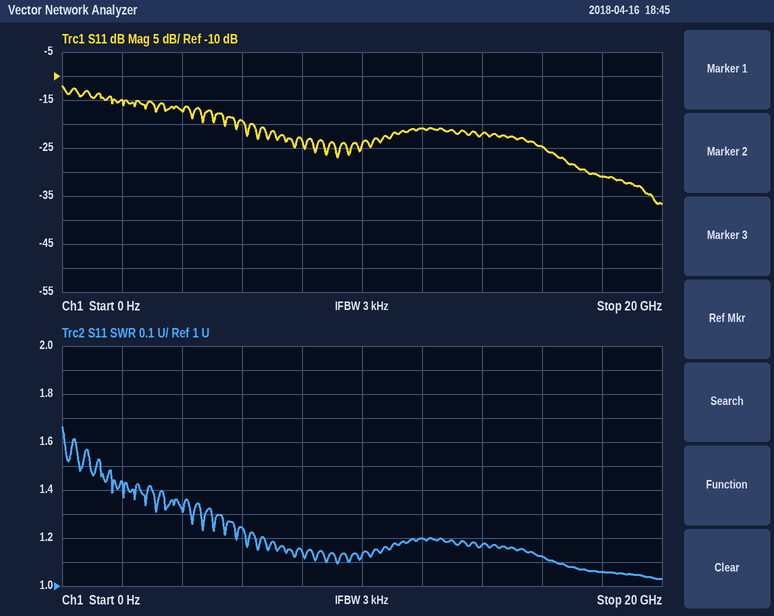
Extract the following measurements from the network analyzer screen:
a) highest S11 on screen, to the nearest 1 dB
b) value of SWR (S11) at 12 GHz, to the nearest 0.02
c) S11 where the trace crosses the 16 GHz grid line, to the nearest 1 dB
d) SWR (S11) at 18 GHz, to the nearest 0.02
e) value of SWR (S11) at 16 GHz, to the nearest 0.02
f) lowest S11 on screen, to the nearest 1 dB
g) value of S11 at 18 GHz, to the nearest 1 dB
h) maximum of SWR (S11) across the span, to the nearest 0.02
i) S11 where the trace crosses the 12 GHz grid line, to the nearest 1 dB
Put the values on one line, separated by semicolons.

-12 dB; 1.20; -25 dB; 1.06; 1.12; -37 dB; -31 dB; 1.66; -21 dB
